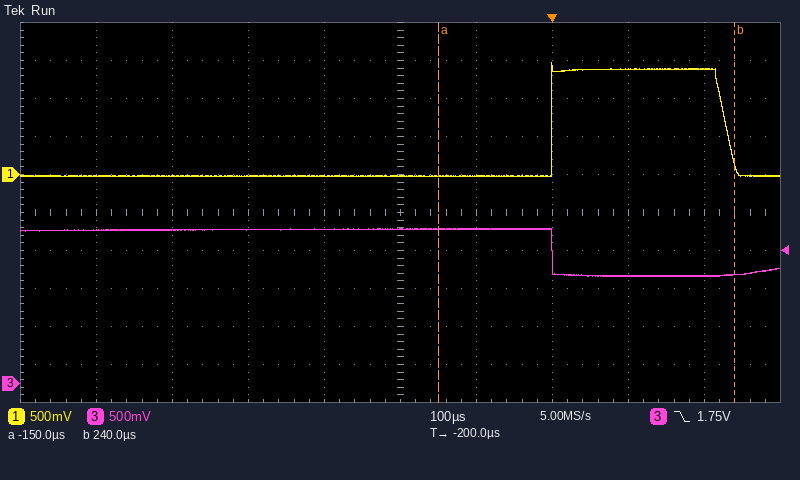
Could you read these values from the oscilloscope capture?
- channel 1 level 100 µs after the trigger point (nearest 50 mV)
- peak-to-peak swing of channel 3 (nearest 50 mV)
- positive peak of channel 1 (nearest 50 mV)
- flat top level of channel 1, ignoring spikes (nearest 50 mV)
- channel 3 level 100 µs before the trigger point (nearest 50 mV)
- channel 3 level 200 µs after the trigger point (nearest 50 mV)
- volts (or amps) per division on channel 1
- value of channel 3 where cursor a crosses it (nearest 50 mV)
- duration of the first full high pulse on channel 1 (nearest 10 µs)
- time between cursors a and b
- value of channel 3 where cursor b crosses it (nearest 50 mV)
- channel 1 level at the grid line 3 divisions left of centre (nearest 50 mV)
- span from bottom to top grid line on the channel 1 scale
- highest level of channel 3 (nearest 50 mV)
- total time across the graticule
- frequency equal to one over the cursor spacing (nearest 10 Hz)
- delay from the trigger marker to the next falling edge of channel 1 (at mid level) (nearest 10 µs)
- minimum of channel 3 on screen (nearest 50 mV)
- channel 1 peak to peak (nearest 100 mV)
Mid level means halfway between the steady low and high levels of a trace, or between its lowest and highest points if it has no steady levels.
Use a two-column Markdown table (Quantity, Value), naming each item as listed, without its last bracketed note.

| Quantity | Value |
|---|---|
| channel 1 level 100 µs after the trigger point | 1.40 V |
| peak-to-peak swing of channel 3 | 650 mV |
| positive peak of channel 1 | 1.45 V |
| flat top level of channel 1, ignoring spikes | 1.40 V |
| channel 3 level 100 µs before the trigger point | 2.05 V |
| channel 3 level 200 µs after the trigger point | 1.40 V |
| volts (or amps) per division on channel 1 | 500 mV |
| value of channel 3 where cursor a crosses it | 2.05 V |
| duration of the first full high pulse on channel 1 | 230 µs |
| time between cursors a and b | 390 µs |
| value of channel 3 where cursor b crosses it | 1.45 V |
| channel 1 level at the grid line 3 divisions left of centre | 0 mV |
| span from bottom to top grid line on the channel 1 scale | 5 V |
| highest level of channel 3 | 2.05 V |
| total time across the graticule | 1 ms |
| frequency equal to one over the cursor spacing | 2.56 kHz |
| delay from the trigger marker to the next falling edge of channel 1 (at mid level) | 230 µs |
| minimum of channel 3 on screen | 1.40 V |
| channel 1 peak to peak | 1.50 V |
